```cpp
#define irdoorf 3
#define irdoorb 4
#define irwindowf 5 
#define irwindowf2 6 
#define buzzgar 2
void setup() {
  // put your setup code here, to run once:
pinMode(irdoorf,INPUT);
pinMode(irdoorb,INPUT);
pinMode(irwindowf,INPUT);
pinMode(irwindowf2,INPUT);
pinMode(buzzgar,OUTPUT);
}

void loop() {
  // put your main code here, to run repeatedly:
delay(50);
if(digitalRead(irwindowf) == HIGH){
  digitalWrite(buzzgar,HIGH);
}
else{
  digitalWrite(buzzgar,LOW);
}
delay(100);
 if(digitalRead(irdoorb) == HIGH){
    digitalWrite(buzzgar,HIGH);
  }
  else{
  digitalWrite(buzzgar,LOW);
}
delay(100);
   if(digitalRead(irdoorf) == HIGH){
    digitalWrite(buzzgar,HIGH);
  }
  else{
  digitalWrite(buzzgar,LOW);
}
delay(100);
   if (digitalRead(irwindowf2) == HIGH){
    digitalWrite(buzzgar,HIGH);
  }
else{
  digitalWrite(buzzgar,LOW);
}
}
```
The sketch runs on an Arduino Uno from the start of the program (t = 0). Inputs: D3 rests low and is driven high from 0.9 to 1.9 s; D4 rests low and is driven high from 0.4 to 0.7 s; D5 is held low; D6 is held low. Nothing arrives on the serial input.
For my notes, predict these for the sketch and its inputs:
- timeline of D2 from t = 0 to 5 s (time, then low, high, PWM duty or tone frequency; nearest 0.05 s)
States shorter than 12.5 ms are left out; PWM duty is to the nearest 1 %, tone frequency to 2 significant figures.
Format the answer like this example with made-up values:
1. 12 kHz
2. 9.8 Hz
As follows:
1. 0 s low; 0.5 s high; 0.6 s low; 0.95 s high; 1.05 s low; 1.3 s high; 1.4 s low; 1.65 s high; 1.75 s low
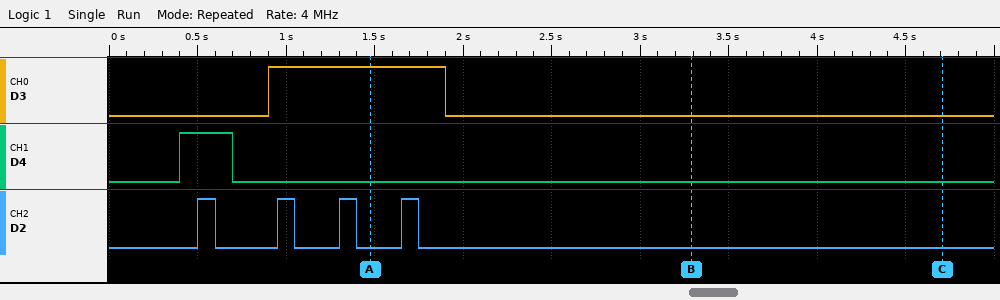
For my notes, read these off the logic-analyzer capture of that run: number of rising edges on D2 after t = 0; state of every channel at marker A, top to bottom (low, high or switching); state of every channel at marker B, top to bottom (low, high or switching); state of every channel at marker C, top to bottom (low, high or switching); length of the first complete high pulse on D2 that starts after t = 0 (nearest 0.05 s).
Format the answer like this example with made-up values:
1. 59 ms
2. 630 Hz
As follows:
1. 4
2. D3 high, D4 low, D2 low
3. D3 low, D4 low, D2 low
4. D3 low, D4 low, D2 low
5. 0.10 s
